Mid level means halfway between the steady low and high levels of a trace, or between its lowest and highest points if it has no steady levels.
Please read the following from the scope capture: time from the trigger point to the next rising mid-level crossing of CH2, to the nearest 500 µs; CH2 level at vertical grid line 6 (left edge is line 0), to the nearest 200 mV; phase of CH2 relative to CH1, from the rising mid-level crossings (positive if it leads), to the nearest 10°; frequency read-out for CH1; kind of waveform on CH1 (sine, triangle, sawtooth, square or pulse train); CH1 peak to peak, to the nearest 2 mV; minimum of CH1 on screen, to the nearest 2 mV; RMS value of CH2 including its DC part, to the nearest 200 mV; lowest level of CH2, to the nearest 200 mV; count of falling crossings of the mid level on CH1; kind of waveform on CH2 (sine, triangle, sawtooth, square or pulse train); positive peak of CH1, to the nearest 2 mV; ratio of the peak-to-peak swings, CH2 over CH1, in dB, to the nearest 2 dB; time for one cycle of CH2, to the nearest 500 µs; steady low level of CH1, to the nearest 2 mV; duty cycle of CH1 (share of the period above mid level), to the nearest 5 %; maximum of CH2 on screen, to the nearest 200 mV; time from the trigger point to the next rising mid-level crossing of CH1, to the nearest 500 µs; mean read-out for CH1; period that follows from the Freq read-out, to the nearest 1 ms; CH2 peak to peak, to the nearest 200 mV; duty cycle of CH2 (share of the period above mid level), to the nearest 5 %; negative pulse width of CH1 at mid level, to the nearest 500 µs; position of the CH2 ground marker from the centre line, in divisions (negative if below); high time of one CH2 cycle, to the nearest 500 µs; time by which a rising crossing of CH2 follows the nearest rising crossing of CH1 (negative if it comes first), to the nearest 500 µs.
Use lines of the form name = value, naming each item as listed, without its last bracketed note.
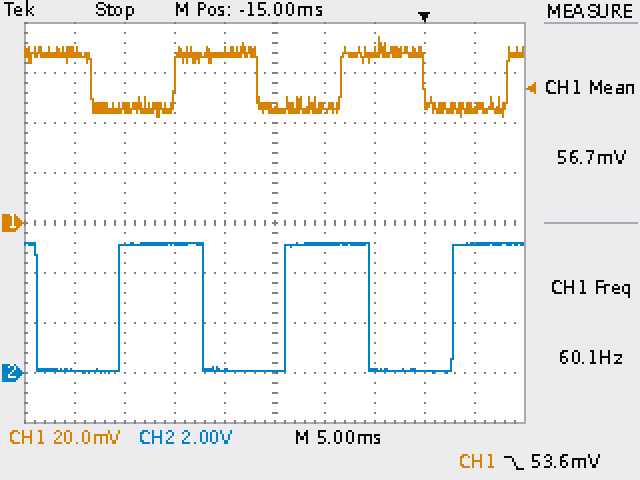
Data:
time from the trigger point to the next rising mid-level crossing of CH2, to the nearest 500 µs = 3.0 ms
CH2 level at vertical grid line 6 (left edge is line 0), to the nearest 200 mV = 5.2 V
phase of CH2 relative to CH1, from the rising mid-level crossings (positive if it leads), to the nearest 10° = +120°
frequency read-out for CH1 = 60.1 Hz
kind of waveform on CH1 = square
CH1 peak to peak, to the nearest 2 mV = 32 mV
minimum of CH1 on screen, to the nearest 2 mV = 42 mV
RMS value of CH2 including its DC part, to the nearest 200 mV = 3.6 V
lowest level of CH2, to the nearest 200 mV = 0.0 V
count of falling crossings of the mid level on CH1 = 3
kind of waveform on CH2 = square
positive peak of CH1, to the nearest 2 mV = 74 mV
ratio of the peak-to-peak swings, CH2 over CH1, in dB, to the nearest 2 dB = 44 dB
time for one cycle of CH2, to the nearest 500 µs = 16.5 ms
steady low level of CH1, to the nearest 2 mV = 46 mV
duty cycle of CH1 (share of the period above mid level), to the nearest 5 % = 50 %
maximum of CH2 on screen, to the nearest 200 mV = 5.2 V
time from the trigger point to the next rising mid-level crossing of CH1, to the nearest 500 µs = 8.5 ms
mean read-out for CH1 = 56.7 mV
period that follows from the Freq read-out, to the nearest 1 ms = 17 ms
CH2 peak to peak, to the nearest 200 mV = 5.2 V
duty cycle of CH2 (share of the period above mid level), to the nearest 5 % = 50 %
negative pulse width of CH1 at mid level, to the nearest 500 µs = 8.5 ms
position of the CH2 ground marker from the centre line, in divisions = -3.0 div
high time of one CH2 cycle, to the nearest 500 µs = 8.5 ms
time by which a rising crossing of CH2 follows the nearest rising crossing of CH1 (negative if it comes first), to the nearest 500 µs = -5.5 ms
